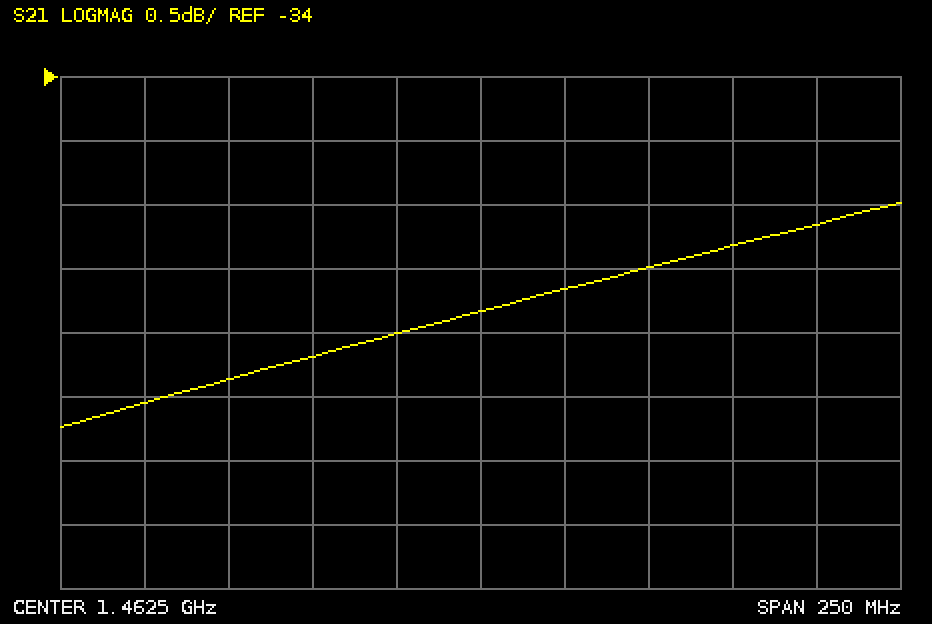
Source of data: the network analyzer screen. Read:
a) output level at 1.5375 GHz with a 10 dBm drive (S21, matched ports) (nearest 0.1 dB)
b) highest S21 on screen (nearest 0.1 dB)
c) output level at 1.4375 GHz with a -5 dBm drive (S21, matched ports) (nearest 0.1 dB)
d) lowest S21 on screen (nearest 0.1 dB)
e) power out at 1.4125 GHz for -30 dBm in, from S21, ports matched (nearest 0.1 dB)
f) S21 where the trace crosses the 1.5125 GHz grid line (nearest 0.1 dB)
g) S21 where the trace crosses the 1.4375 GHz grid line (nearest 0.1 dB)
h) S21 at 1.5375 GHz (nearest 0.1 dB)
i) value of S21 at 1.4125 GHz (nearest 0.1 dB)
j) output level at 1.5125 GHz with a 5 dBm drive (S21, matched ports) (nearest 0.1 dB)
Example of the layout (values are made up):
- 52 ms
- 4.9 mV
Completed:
- -25.3 dBm
- -35.0 dB
- -41.0 dBm
- -36.7 dB
- -66.2 dBm
- -35.5 dB
- -36.0 dB
- -35.3 dB
- -36.2 dB
- -30.5 dBm
